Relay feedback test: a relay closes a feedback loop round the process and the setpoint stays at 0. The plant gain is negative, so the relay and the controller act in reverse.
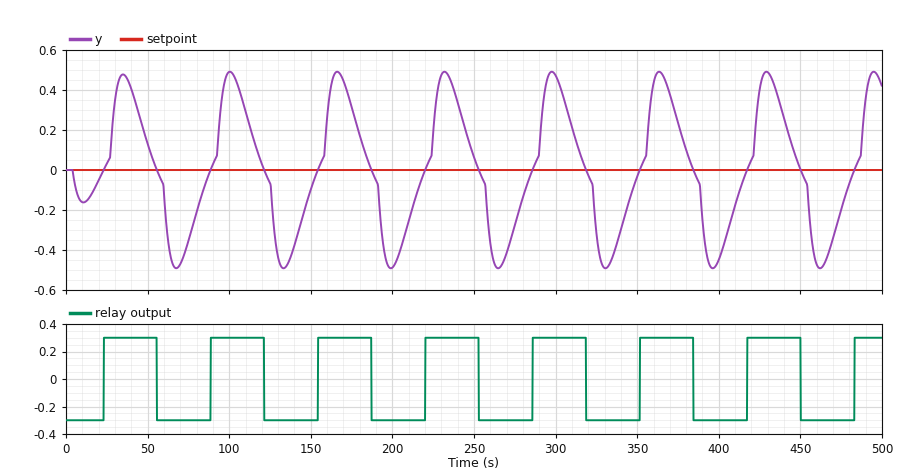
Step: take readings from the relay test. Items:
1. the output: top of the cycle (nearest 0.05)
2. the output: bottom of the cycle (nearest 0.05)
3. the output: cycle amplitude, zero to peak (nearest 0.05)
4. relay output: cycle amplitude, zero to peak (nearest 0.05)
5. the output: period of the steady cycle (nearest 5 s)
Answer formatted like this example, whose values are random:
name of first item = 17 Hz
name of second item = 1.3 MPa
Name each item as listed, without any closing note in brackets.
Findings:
the output: top of the cycle = 0.50
the output: bottom of the cycle = -0.50
the output: cycle amplitude, zero to peak = 0.50
relay output: cycle amplitude, zero to peak = 0.30
the output: period of the steady cycle = 65 s
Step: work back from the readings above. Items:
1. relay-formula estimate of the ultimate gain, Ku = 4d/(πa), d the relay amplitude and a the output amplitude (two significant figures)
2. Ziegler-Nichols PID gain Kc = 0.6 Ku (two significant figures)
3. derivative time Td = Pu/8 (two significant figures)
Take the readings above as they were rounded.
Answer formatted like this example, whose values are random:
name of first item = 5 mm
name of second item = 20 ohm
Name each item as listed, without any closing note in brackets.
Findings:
relay-formula estimate of the ultimate gain, Ku = 4d/(πa), d the relay amplitude and a the output amplitude = 0.76
Ziegler-Nichols PID gain Kc = 0.6 Ku = 0.46
derivative time Td = Pu/8 = 8.1 s
